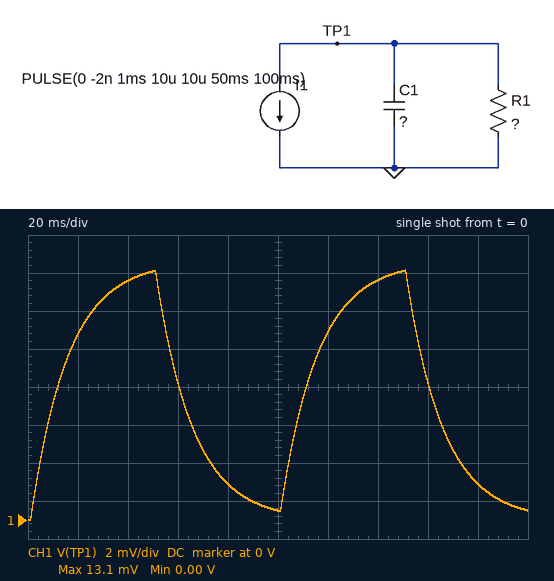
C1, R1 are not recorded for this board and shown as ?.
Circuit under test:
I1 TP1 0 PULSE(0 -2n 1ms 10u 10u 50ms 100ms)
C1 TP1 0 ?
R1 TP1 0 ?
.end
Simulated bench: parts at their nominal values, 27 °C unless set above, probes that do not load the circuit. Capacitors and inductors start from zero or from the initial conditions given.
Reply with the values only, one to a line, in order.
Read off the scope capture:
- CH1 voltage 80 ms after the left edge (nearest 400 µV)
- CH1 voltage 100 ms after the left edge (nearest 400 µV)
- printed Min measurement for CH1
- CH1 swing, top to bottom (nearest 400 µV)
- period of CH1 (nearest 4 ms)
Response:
2.0 mV
400 µV
0.00 V
13.2 mV
100 ms
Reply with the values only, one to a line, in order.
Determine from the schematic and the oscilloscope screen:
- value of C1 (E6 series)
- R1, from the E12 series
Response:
2.2 nF
6.8 MΩ
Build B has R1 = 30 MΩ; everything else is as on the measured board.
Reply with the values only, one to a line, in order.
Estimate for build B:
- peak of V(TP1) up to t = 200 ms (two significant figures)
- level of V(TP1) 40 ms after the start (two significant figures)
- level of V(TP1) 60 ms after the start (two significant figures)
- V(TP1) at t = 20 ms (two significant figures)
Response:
39 mV
27 mV
28 mV
15 mV
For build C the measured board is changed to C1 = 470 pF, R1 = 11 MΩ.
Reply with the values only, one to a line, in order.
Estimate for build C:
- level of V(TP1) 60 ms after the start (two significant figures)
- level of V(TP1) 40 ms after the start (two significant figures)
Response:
3.9 mV
22 mV
